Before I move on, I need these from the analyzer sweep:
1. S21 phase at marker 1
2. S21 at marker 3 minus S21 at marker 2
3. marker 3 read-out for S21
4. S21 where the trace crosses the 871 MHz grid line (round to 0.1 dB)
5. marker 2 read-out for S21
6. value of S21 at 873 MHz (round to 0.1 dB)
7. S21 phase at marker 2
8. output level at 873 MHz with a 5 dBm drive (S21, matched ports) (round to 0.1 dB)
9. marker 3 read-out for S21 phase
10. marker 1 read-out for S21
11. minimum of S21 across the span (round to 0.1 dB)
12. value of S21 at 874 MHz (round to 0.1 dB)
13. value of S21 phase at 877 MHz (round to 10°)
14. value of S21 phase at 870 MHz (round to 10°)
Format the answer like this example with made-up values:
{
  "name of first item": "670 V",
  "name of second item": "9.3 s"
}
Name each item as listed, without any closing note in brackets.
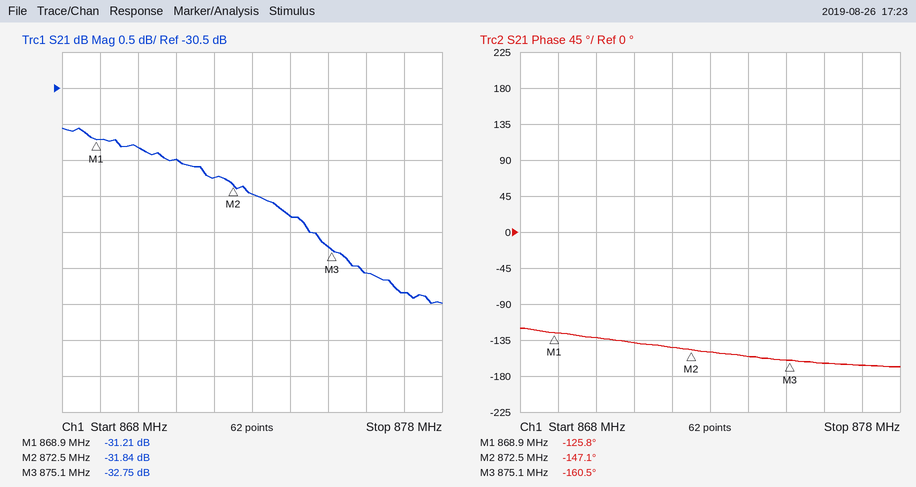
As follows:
{
  "S21 phase at marker 1": "-125.8°",
  "S21 at marker 3 minus S21 at marker 2": "-0.91 dB",
  "marker 3 read-out for S21": "-32.75 dB",
  "S21 where the trace crosses the 871 MHz grid line": "-31.5 dB",
  "marker 2 read-out for S21": "-31.84 dB",
  "value of S21 at 873 MHz": "-32.0 dB",
  "S21 phase at marker 2": "-147.1°",
  "output level at 873 MHz with a 5 dBm drive (S21, matched ports)": "-27.0 dBm",
  "marker 3 read-out for S21 phase": "-160.5°",
  "marker 1 read-out for S21": "-31.21 dB",
  "minimum of S21 across the span": "-33.5 dB",
  "value of S21 at 874 MHz": "-32.3 dB",
  "value of S21 phase at 877 MHz": "-170°",
  "value of S21 phase at 870 MHz": "-130°"
}
